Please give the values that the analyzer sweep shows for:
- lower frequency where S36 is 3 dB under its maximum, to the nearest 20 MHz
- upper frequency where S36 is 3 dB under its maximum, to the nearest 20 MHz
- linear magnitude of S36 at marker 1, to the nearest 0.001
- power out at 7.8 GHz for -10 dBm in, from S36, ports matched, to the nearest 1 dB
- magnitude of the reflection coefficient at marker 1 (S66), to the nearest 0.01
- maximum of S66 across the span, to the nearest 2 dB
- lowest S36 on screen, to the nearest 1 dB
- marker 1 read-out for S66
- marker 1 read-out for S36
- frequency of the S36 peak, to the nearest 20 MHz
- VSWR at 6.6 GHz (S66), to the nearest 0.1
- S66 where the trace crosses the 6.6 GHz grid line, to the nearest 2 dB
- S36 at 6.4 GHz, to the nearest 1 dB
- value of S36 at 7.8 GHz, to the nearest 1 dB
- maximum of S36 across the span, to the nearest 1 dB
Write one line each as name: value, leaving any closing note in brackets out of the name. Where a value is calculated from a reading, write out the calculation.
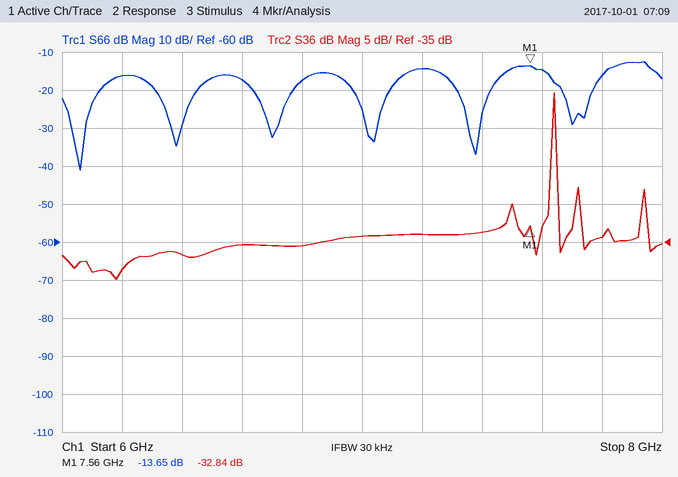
lower frequency where S36 is 3 dB under its maximum, to the nearest 20 MHz: 7.64 GHz
upper frequency where S36 is 3 dB under its maximum, to the nearest 20 MHz: 7.64 GHz
linear magnitude of S36 at marker 1, to the nearest 0.001: 10^(-32.84/20) ≈ 0.023
power out at 7.8 GHz for -10 dBm in, from S36, ports matched, to the nearest 1 dB: -10 dBm + (-34 dB) = -44 dBm
magnitude of the reflection coefficient at marker 1 (S66), to the nearest 0.01: 10^(-13.65/20) ≈ 0.21
maximum of S66 across the span, to the nearest 2 dB: -12 dB
lowest S36 on screen, to the nearest 1 dB: -40 dB
marker 1 read-out for S66: -13.65 dB
marker 1 read-out for S36: -32.84 dB
frequency of the S36 peak, to the nearest 20 MHz: 7.64 GHz
VSWR at 6.6 GHz (S66), to the nearest 0.1: |Γ| = 10^(-18/20) = 0.1259; VSWR = (1 + 0.1259)/(1 − 0.1259) ≈ 1.3
S66 where the trace crosses the 6.6 GHz grid line, to the nearest 2 dB: -18 dB
S36 at 6.4 GHz, to the nearest 1 dB: -37 dB
value of S36 at 7.8 GHz, to the nearest 1 dB: -34 dB
maximum of S36 across the span, to the nearest 1 dB: -15 dB
